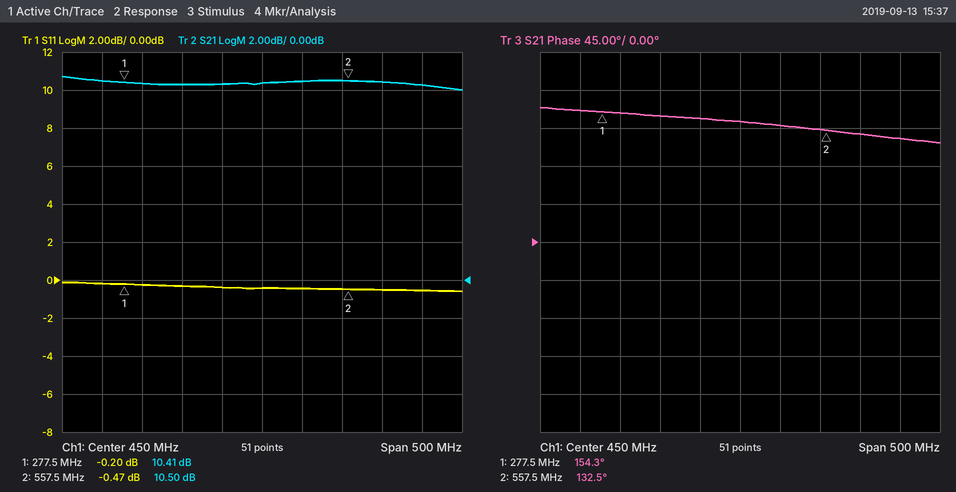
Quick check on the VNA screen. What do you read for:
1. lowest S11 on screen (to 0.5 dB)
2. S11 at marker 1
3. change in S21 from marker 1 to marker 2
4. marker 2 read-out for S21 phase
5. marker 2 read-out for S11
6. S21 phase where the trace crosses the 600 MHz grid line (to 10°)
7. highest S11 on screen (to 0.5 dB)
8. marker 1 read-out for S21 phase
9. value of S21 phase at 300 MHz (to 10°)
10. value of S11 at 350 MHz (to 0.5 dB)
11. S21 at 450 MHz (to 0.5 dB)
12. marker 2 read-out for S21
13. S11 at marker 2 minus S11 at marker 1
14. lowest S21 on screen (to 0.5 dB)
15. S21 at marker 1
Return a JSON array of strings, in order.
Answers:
["-0.5 dB", "-0.20 dB", "0.09 dB", "132.5°", "-0.47 dB", "130°", "0.0 dB", "154.3°", "150°", "-0.5 dB", "10.5 dB", "10.50 dB", "-0.27 dB", "10.0 dB", "10.41 dB"]
